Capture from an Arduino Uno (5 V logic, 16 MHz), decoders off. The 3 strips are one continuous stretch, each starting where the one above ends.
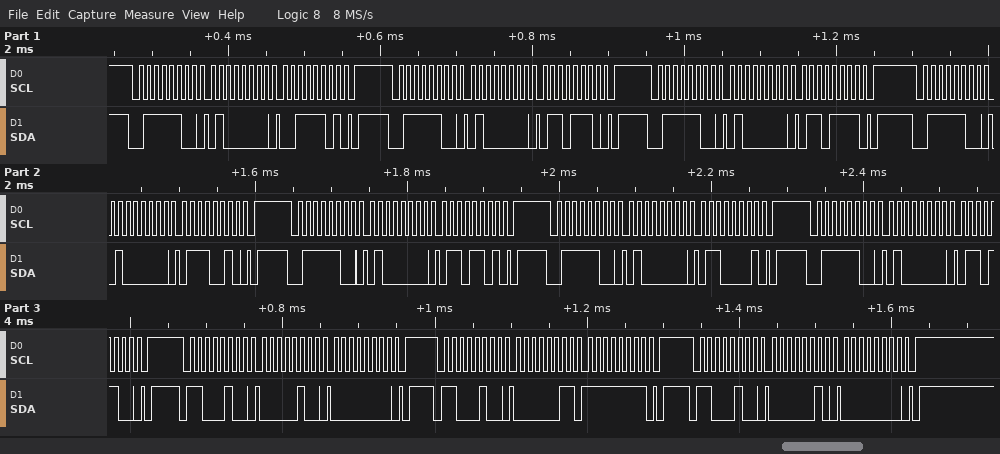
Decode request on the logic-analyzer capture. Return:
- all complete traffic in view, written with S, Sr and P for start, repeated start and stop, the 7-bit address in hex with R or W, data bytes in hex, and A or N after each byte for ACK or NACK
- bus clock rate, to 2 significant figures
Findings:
S 3EW A 40 A 3D A P S 3EW A 40 A 6E A P S 3EW A 40 A 6F A P S 3EW A 40 A 72 A P S 3EW A 40 A 6D A P S 3EW A 40 A 61 A P S 3EW A 40 A 6C A P S 62W A 04 A 00 A P S 62W A 03 A FF A P S 62W A 02 A 00 A P
100 kHz
